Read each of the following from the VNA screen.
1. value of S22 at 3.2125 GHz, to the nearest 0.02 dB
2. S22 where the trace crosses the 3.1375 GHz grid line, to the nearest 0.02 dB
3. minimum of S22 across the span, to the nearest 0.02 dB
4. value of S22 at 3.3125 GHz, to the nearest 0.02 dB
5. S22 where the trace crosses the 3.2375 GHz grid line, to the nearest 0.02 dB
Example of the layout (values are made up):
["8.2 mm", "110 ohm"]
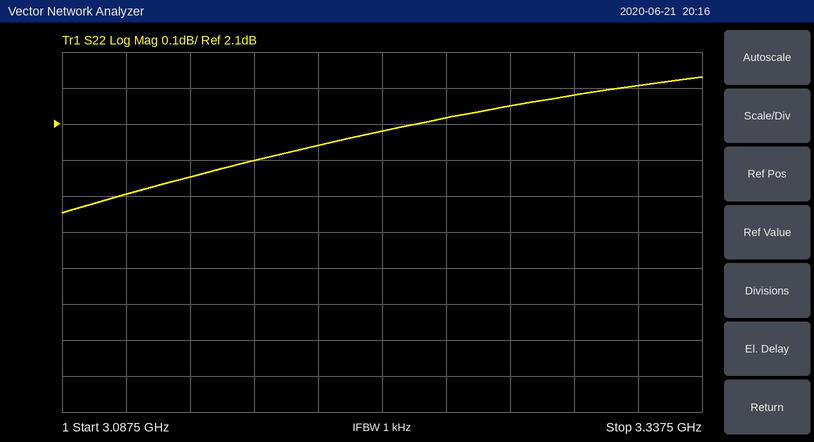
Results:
["2.08 dB", "1.96 dB", "1.86 dB", "2.20 dB", "2.12 dB"]
